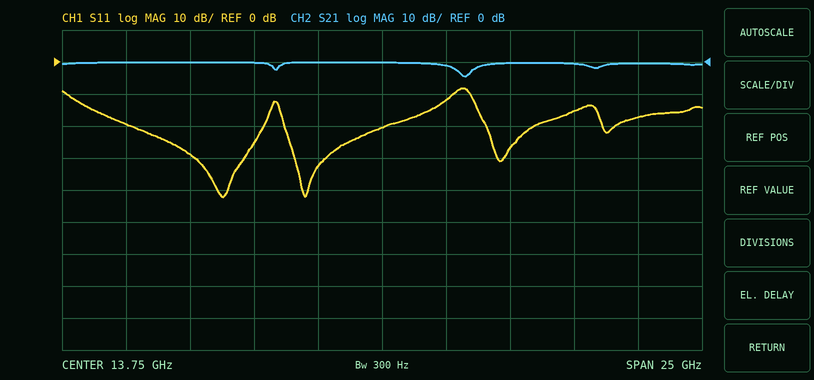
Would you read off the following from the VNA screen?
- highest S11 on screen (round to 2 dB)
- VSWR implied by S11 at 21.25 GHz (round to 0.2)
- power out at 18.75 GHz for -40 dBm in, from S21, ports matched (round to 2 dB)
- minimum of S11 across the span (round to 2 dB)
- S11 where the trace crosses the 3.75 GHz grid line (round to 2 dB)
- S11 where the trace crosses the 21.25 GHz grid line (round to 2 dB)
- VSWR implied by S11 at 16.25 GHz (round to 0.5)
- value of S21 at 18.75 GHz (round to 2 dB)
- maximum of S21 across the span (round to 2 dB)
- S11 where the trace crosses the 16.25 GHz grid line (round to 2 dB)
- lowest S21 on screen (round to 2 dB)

-8 dB
1.4
-40 dBm
-42 dB
-20 dB
-16 dB
1.5
0 dB
0 dB
-12 dB
-4 dB
